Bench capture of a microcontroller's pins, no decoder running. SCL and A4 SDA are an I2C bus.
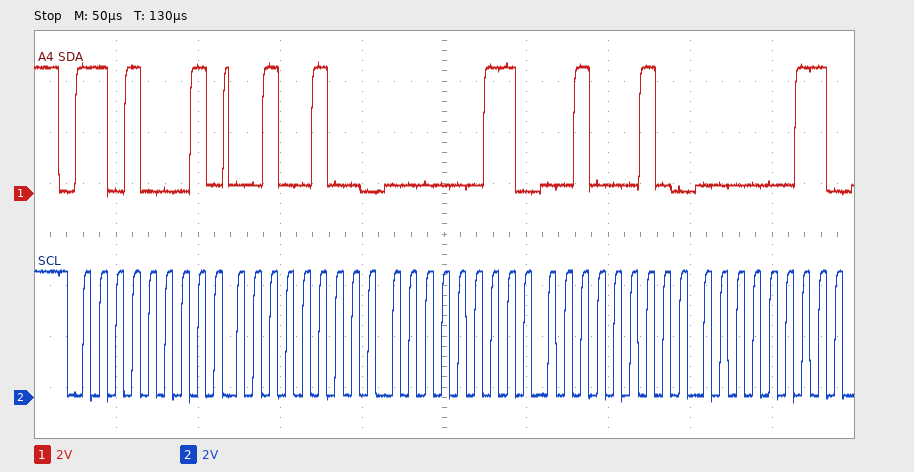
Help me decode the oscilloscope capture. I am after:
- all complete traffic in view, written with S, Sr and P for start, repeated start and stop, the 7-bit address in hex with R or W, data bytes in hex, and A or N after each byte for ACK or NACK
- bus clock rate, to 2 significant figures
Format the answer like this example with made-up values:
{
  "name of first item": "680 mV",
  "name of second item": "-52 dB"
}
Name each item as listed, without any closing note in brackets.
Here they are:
{
  "all complete traffic in view, written with S, Sr and P for start, repeated start and stop, the 7-bit address in hex with R or W, data bytes in hex, and A or N after each byte for ACK or NACK": "S 68R A 24 A 03 A 22 A 03 A",
  "bus clock rate, to 2 significant figures": "100 kHz"
}
